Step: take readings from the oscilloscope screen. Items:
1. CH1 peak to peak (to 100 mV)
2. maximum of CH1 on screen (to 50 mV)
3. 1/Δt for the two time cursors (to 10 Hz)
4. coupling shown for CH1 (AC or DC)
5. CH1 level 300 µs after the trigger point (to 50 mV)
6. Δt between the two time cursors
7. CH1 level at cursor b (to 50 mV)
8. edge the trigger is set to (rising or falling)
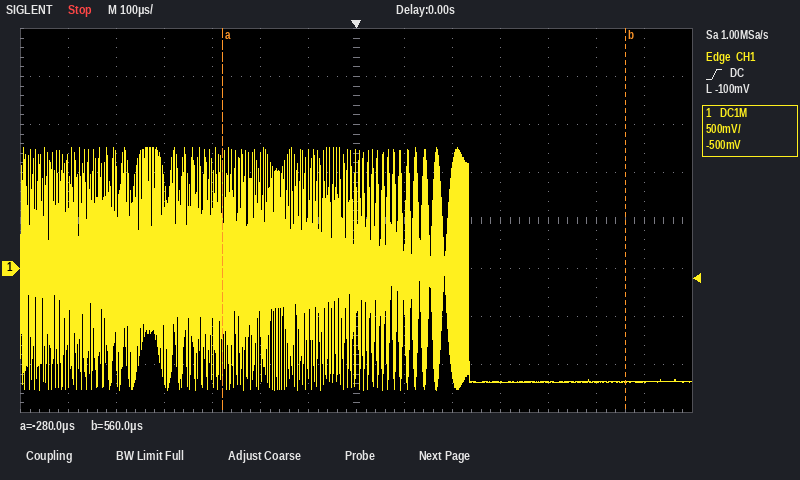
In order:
2.50 V
1.25 V
1.19 kHz
DC
-1.20 V
840 µs
-1.20 V
rising
